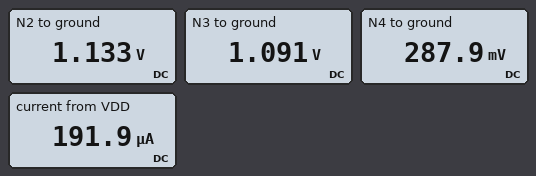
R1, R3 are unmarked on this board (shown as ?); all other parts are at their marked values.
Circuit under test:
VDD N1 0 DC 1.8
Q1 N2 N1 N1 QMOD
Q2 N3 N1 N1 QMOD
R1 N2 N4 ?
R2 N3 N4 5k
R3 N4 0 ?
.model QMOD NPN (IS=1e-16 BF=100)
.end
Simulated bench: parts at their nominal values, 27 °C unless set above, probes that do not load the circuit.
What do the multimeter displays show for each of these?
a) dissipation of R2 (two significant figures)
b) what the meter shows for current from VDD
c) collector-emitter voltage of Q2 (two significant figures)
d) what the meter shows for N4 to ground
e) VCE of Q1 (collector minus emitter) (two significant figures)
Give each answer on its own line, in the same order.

130 µW
191.9 µA
-710 mV
287.9 mV
-670 mV
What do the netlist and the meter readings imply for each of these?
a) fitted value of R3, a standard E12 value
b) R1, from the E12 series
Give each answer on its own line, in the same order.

1.5 kΩ
27 kΩ
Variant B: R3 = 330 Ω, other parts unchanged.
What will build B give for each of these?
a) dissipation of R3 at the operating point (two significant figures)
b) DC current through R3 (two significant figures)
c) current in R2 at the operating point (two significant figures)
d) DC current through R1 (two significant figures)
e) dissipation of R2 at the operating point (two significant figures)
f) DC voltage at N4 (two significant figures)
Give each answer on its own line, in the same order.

19 µW
240 µA
200 µA
39 µA
200 µW
79 mV
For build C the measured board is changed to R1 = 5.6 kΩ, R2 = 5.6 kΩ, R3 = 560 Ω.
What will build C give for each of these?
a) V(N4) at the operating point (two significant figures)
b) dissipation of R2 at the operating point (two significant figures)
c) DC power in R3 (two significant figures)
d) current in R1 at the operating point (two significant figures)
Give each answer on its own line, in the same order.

180 mV
150 µW
59 µW
160 µA
